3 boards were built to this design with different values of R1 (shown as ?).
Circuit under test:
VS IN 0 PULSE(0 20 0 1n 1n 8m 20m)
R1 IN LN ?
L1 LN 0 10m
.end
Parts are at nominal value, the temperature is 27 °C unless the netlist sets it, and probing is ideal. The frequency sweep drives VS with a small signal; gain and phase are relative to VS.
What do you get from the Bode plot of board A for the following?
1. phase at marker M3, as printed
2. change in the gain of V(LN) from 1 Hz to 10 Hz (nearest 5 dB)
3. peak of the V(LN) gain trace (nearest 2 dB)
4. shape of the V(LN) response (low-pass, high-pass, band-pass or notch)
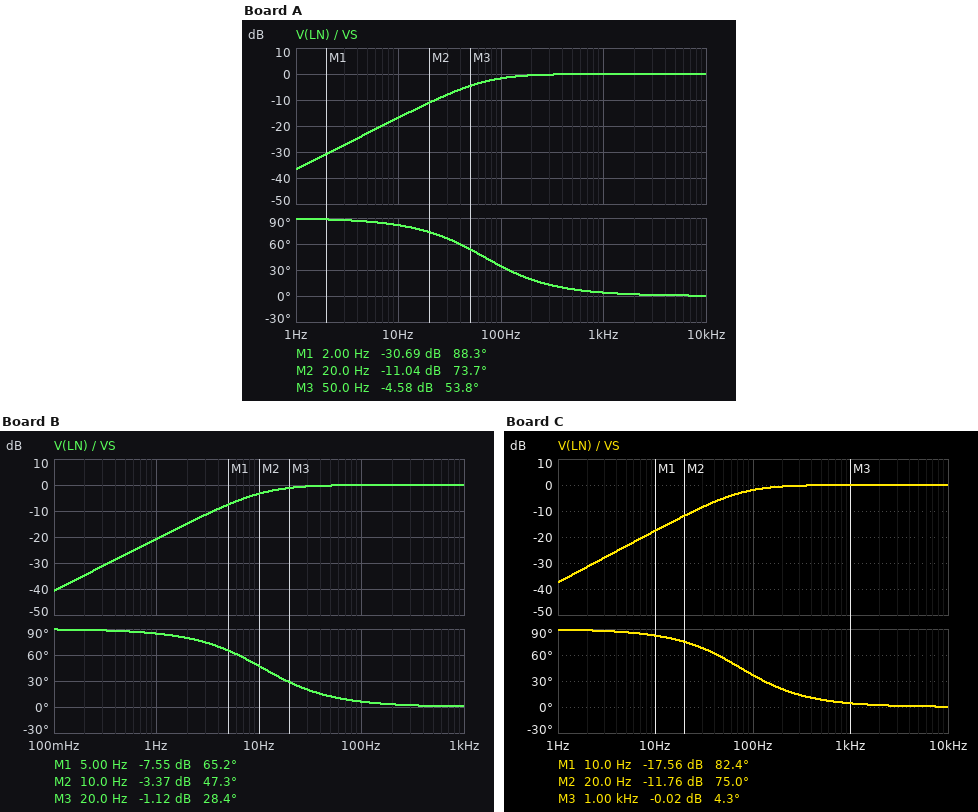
53.8 deg
20 dB
0 dB
high-pass
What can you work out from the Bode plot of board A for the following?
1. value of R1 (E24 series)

4.3 Ω
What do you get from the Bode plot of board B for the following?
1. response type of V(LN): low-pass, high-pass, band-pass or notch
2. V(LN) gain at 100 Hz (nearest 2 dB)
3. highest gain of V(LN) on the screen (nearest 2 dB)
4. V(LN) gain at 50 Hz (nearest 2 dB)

high-pass
0 dB
0 dB
0 dB
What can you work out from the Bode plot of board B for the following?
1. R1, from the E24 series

0.68 Ω
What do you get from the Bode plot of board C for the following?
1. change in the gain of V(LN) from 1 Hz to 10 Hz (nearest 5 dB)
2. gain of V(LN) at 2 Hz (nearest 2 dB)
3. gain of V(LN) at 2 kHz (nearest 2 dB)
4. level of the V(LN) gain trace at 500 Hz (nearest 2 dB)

20 dB
-32 dB
0 dB
0 dB
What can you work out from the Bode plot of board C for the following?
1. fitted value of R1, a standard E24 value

4.7 Ω
